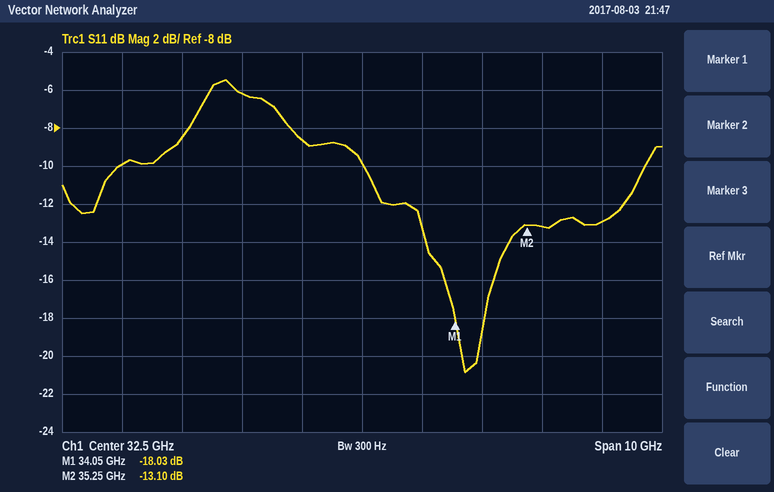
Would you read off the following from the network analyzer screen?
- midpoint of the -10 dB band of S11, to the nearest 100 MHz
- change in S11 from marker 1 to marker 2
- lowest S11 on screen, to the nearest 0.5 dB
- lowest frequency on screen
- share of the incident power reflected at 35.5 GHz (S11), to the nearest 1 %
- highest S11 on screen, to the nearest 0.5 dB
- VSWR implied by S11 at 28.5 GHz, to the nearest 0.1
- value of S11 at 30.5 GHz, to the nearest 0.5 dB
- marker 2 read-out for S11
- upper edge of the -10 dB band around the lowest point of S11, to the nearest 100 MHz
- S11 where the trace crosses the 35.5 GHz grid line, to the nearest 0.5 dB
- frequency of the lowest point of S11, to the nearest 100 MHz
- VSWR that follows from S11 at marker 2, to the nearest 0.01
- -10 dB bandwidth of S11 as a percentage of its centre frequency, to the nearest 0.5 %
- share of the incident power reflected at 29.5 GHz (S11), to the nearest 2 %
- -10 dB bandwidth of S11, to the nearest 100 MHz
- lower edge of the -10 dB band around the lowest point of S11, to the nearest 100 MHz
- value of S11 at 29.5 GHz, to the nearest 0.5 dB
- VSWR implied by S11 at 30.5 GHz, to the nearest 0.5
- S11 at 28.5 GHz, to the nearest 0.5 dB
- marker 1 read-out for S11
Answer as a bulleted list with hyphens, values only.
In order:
- 34.9 GHz
- 4.93 dB
- -21.0 dB
- 27.5 GHz
- 5 %
- -5.5 dB
- 1.9
- -6.0 dB
- -13.10 dB
- 37.2 GHz
- -13.0 dB
- 34.2 GHz
- 1.57
- 13.5 %
- 14 %
- 4.7 GHz
- 32.5 GHz
- -8.5 dB
- 3.0
- -10.0 dB
- -18.03 dB
